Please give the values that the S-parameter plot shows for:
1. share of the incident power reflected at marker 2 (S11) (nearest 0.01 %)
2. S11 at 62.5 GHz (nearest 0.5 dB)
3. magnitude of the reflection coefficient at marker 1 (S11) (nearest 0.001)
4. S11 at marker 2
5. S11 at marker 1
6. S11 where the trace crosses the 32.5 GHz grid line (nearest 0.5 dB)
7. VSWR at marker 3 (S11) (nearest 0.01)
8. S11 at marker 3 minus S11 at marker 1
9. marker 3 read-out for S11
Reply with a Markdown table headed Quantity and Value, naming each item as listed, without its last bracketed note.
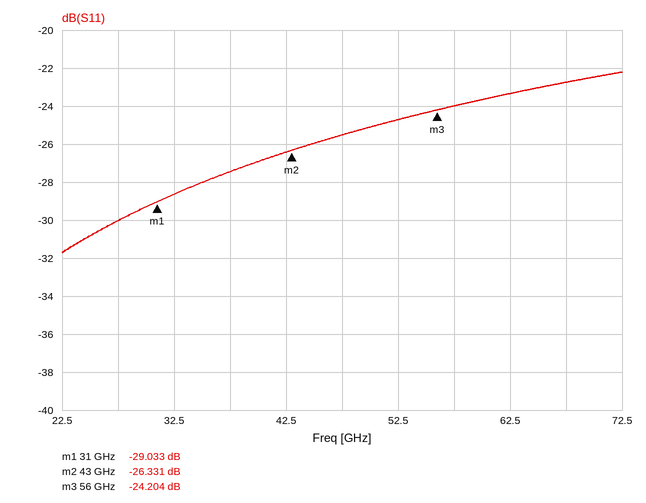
| Quantity | Value |
|---|---|
| share of the incident power reflected at marker 2 (S11) | 0.23 % |
| S11 at 62.5 GHz | -23.5 dB |
| magnitude of the reflection coefficient at marker 1 (S11) | 0.035 |
| S11 at marker 2 | -26.331 dB |
| S11 at marker 1 | -29.033 dB |
| S11 where the trace crosses the 32.5 GHz grid line | -28.5 dB |
| VSWR at marker 3 (S11) | 1.13 |
| S11 at marker 3 minus S11 at marker 1 | 4.829 dB |
| marker 3 read-out for S11 | -24.204 dB |
